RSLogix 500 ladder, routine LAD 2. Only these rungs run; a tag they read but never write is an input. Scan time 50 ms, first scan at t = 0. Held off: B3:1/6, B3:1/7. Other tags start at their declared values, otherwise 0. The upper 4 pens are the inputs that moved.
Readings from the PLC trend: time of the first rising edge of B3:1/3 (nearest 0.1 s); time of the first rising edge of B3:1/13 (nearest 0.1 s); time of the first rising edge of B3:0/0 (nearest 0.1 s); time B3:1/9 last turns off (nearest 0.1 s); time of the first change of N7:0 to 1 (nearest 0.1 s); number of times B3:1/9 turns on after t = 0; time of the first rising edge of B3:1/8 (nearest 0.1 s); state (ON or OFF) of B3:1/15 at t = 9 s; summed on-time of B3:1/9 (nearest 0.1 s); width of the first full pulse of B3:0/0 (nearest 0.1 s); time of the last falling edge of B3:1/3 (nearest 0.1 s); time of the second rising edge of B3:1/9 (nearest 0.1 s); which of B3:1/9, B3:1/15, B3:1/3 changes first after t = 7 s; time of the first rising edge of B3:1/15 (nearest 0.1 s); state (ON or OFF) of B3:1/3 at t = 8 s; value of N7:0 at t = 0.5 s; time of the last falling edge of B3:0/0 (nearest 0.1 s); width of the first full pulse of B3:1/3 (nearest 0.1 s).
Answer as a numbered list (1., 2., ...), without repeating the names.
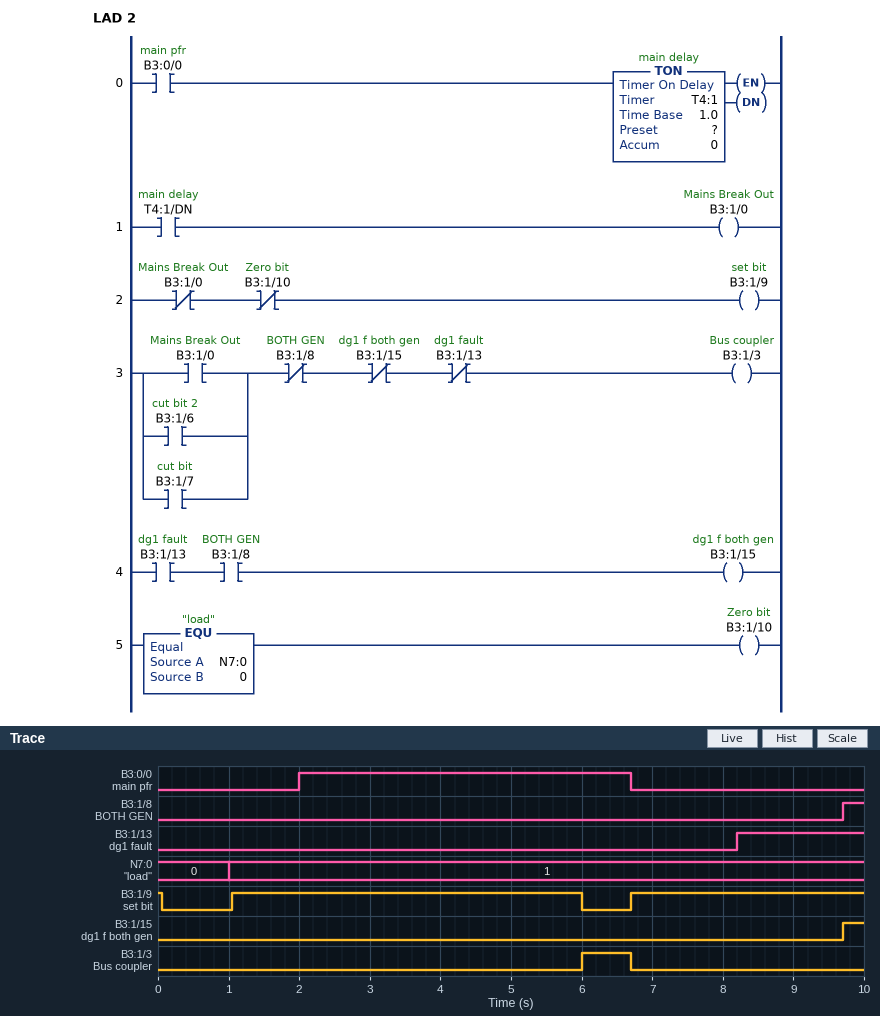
1. 6.0 s
2. 8.2 s
3. 2.0 s
4. 6.0 s
5. 1.0 s
6. 2
7. 9.7 s
8. OFF
9. 8.3 s
10. 4.7 s
11. 6.7 s
12. 6.7 s
13. B3:1/15
14. 9.7 s
15. OFF
16. 0
17. 6.7 s
18. 0.7 s
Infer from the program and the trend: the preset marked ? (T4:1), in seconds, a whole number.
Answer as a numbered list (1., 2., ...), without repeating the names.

1. 4 s
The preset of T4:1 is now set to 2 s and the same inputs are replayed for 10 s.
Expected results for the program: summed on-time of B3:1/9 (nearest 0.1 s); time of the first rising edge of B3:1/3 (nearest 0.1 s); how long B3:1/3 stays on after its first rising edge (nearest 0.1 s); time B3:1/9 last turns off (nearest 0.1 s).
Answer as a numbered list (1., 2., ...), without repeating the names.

1. 6.3 s
2. 4.0 s
3. 2.7 s
4. 4.0 s
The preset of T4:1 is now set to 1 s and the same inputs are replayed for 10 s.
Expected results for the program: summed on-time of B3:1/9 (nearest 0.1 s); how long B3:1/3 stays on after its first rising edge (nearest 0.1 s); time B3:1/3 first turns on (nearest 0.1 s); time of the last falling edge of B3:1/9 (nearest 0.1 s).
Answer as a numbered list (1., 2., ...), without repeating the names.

1. 5.3 s
2. 3.7 s
3. 3.0 s
4. 3.0 s
